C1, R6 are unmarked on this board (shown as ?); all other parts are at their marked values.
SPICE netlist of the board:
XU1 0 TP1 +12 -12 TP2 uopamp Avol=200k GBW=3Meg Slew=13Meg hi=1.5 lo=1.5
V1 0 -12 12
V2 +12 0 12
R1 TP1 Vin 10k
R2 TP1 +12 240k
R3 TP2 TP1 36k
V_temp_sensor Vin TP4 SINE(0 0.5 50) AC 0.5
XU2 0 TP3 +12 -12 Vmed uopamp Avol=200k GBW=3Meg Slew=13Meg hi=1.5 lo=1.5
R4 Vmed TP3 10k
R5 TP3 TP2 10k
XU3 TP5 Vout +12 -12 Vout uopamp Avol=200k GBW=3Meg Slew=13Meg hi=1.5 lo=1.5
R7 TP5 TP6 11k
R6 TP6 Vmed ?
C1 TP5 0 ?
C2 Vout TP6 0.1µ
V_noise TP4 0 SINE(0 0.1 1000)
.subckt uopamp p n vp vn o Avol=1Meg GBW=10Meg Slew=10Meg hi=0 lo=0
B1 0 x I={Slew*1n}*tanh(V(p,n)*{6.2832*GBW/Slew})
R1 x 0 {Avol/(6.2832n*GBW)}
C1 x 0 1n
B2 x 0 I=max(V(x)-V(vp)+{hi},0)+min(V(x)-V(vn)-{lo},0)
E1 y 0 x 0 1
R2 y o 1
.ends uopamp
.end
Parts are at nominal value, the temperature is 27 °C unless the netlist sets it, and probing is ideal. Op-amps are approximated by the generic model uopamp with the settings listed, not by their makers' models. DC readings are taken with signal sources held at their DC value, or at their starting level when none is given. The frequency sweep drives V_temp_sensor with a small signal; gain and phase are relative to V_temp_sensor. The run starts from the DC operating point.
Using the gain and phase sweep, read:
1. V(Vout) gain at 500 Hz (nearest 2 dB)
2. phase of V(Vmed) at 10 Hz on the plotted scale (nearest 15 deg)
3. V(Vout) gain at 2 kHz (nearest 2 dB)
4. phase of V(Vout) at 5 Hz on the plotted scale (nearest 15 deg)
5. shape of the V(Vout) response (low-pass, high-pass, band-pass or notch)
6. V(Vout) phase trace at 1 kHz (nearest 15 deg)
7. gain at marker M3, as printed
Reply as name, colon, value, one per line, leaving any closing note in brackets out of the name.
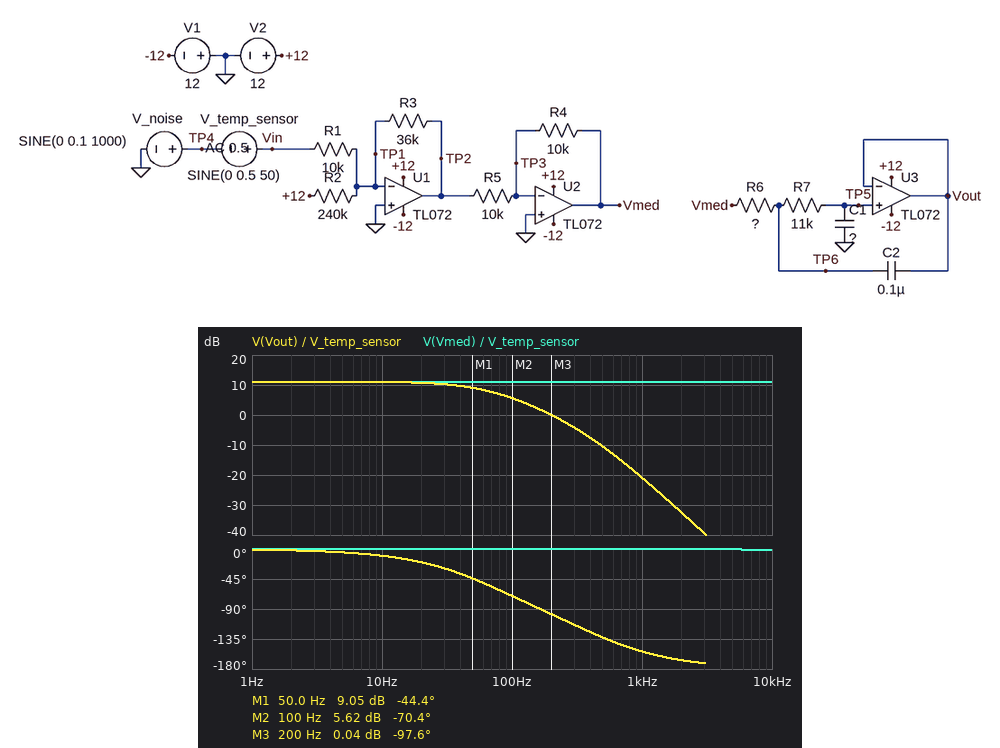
V(Vout) gain at 500 Hz: -10 dB
phase of V(Vmed) at 10 Hz on the plotted scale: 0 deg
V(Vout) gain at 2 kHz: -32 dB
phase of V(Vout) at 5 Hz on the plotted scale: 0 deg
shape of the V(Vout) response: low-pass
V(Vout) phase trace at 1 kHz: -150 deg
gain at marker M3, as printed: 0.04 dB
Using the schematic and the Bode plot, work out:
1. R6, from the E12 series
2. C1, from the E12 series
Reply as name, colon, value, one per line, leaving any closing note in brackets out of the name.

R6, from the E12 series: 4.7 kΩ
C1, from the E12 series: 180 nF
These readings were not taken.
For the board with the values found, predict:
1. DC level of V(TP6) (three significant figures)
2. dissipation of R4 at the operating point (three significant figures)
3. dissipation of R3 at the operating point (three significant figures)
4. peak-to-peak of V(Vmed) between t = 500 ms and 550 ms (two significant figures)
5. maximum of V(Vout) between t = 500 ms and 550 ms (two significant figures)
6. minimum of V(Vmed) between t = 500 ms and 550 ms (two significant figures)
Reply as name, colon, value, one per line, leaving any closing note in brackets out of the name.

DC level of V(TP6): 1.80 V
dissipation of R4 at the operating point: 324 µW
dissipation of R3 at the operating point: 90.0 µW
peak-to-peak of V(Vmed) between t = 500 ms and 550 ms: 4.3 V
maximum of V(Vout) between t = 500 ms and 550 ms: 3.2 V
minimum of V(Vmed) between t = 500 ms and 550 ms: -350 mV
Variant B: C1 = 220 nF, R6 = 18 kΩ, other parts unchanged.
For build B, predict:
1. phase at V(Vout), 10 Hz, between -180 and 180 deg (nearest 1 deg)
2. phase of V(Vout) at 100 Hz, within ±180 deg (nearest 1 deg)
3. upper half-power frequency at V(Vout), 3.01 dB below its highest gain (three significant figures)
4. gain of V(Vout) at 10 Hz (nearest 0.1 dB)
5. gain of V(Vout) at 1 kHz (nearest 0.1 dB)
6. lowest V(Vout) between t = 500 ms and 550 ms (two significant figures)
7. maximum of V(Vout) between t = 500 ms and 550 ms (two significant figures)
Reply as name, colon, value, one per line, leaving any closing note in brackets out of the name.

phase at V(Vout), 10 Hz, between -180 and 180 deg: -22 deg
phase of V(Vout) at 100 Hz, within ±180 deg: -100 deg
upper half-power frequency at V(Vout), 3.01 dB below its highest gain: 27.9 Hz
gain of V(Vout) at 10 Hz: 10.6 dB
gain of V(Vout) at 1 kHz: -33.8 dB
lowest V(Vout) between t = 500 ms and 550 ms: 930 mV
maximum of V(Vout) between t = 500 ms and 550 ms: 2.7 V
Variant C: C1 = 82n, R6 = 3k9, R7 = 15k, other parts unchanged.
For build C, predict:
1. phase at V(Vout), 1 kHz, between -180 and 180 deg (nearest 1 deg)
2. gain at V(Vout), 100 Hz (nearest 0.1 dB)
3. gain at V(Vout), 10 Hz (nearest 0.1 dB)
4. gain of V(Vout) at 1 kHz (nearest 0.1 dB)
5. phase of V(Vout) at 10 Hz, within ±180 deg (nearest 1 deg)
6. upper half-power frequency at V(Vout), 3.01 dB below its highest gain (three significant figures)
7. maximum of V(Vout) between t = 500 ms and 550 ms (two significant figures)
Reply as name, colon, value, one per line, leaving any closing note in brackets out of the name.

phase at V(Vout), 1 kHz, between -180 and 180 deg: -152 deg
gain at V(Vout), 100 Hz: 9.1 dB
gain at V(Vout), 10 Hz: 11.1 dB
gain of V(Vout) at 1 kHz: -15.1 dB
phase of V(Vout) at 10 Hz, within ±180 deg: -6 deg
upper half-power frequency at V(Vout), 3.01 dB below its highest gain: 126 Hz
maximum of V(Vout) between t = 500 ms and 550 ms: 3.5 V
